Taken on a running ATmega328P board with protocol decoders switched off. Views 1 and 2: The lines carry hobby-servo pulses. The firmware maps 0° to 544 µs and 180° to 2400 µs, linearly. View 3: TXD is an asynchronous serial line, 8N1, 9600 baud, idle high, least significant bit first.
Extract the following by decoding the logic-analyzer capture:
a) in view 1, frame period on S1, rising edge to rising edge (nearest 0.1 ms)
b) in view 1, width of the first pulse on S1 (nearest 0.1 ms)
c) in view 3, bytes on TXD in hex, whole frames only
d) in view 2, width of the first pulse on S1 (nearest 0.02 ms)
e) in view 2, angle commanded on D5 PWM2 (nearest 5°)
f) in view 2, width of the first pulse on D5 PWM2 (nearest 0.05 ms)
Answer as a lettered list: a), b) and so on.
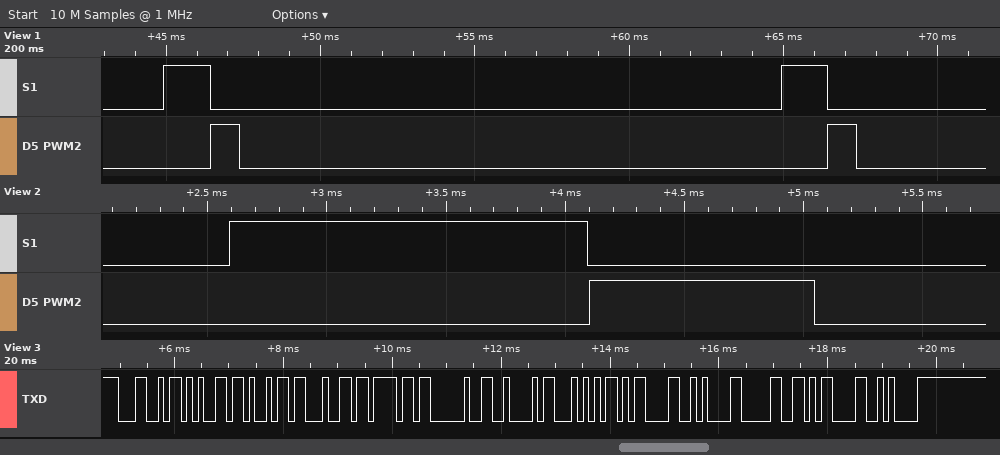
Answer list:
a) 20.0 ms
b) 1.5 ms
c) 4C 65 69 64 6F 20 42 54 0D 0A 30 0D 0A
d) 1.50 ms
e) 40°
f) 0.95 ms
